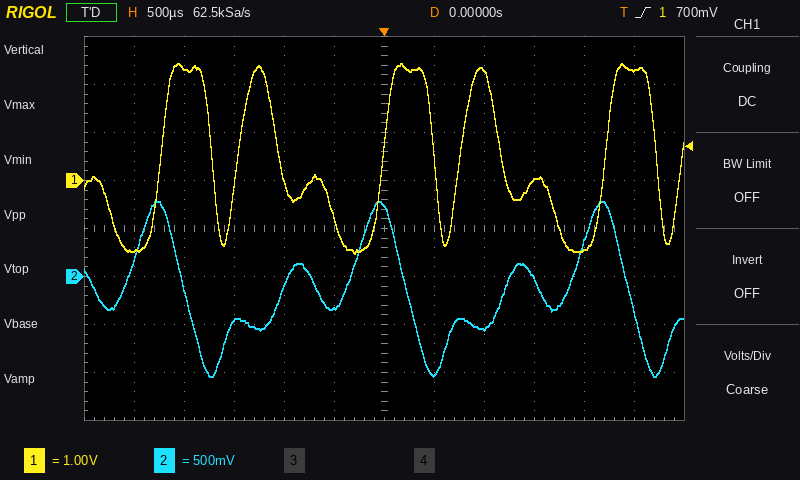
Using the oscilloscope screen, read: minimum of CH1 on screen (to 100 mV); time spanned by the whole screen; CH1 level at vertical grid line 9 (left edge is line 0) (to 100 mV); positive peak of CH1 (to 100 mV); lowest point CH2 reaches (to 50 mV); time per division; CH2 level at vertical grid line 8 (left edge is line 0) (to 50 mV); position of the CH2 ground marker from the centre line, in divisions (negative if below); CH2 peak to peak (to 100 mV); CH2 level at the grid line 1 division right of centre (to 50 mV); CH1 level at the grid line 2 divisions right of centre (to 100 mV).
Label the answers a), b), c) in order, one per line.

a) -1.5 V
b) 6 ms
c) 0.0 V
d) 2.4 V
e) -1.05 V
f) 500 µs
g) -550 mV
h) -1.0 div
i) 1.80 V
j) -1.00 V
k) 2.3 V
